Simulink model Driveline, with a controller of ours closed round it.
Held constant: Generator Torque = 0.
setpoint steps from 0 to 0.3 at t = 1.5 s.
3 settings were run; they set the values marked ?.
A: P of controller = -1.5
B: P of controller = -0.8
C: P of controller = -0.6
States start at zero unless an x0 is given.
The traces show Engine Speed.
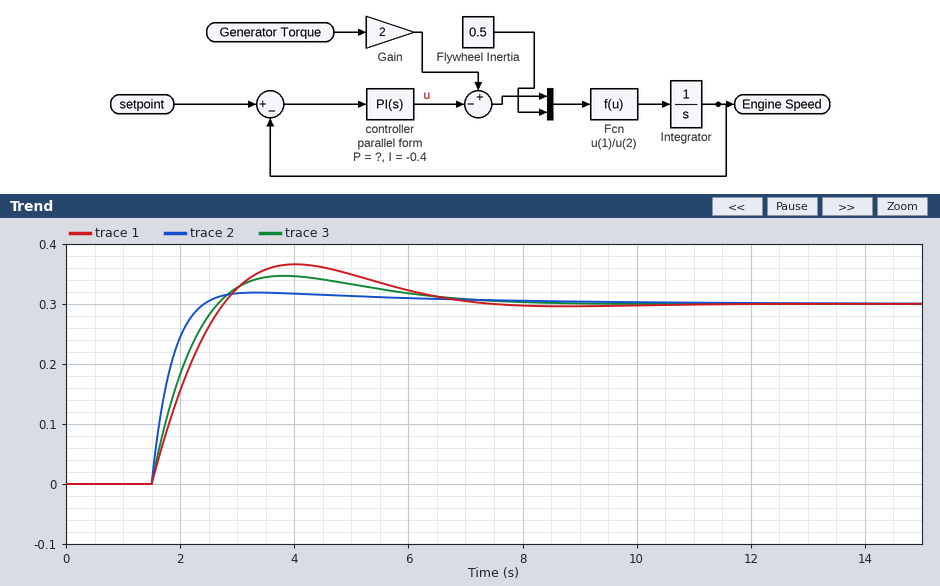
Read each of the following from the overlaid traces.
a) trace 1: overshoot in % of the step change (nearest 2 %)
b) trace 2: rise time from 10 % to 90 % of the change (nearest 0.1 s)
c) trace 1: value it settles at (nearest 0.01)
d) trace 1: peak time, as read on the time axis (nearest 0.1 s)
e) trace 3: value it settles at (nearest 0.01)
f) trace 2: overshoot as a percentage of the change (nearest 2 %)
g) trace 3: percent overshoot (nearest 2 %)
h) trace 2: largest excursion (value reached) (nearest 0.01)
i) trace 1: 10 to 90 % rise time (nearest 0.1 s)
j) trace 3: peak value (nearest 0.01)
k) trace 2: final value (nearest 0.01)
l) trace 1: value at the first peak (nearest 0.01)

22 %
0.6 s
0.30
4.0 s
0.30
6 %
16 %
0.32
1.0 s
0.35
0.30
0.37
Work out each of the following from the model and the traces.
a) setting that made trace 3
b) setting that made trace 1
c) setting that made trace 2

B
C
A
